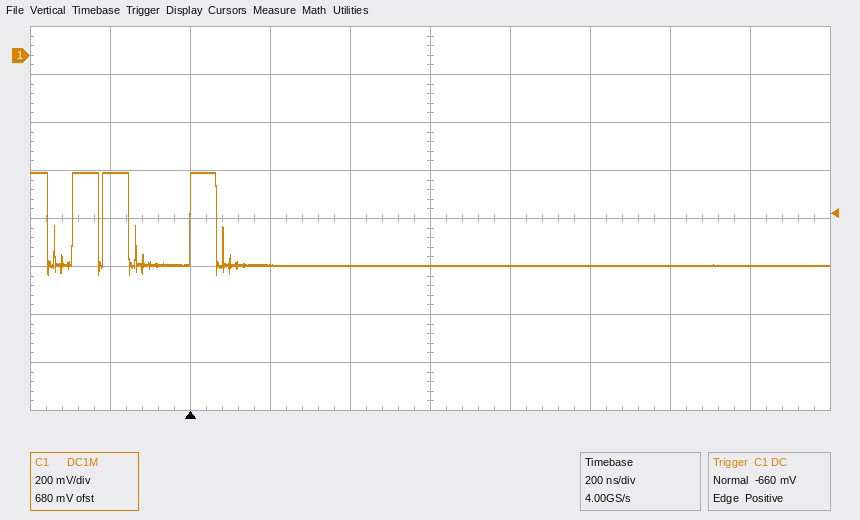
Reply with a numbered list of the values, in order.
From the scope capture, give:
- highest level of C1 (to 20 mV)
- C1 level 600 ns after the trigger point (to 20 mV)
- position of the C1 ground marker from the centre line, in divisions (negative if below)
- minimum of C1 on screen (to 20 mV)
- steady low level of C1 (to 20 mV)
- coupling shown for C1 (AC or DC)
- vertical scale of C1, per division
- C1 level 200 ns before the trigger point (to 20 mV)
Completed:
1. -480 mV
2. -880 mV
3. +3.4 div
4. -920 mV
5. -880 mV
6. DC
7. 200 mV
8. -480 mV
